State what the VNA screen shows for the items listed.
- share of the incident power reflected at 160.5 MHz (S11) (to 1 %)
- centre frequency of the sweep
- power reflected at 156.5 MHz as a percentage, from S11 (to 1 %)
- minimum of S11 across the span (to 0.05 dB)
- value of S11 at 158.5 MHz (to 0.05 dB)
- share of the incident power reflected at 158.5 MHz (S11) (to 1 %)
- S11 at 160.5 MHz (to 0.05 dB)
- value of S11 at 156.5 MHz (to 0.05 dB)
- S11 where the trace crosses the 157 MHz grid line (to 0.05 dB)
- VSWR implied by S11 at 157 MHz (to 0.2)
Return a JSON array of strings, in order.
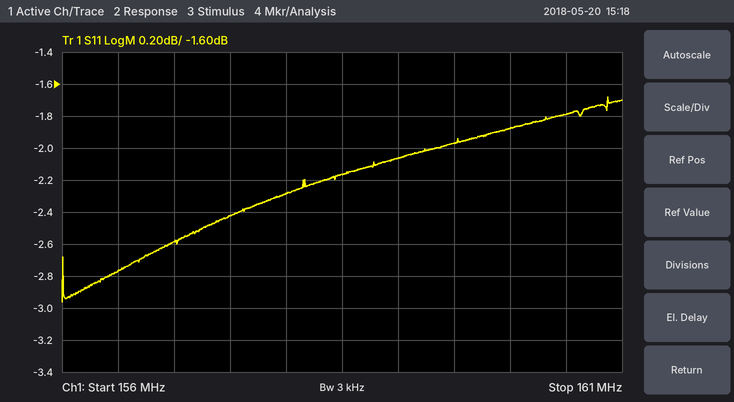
["66 %", "158.5 MHz", "53 %", "-2.95 dB", "-2.15 dB", "61 %", "-1.80 dB", "-2.75 dB", "-2.60 dB", "6.8"]
